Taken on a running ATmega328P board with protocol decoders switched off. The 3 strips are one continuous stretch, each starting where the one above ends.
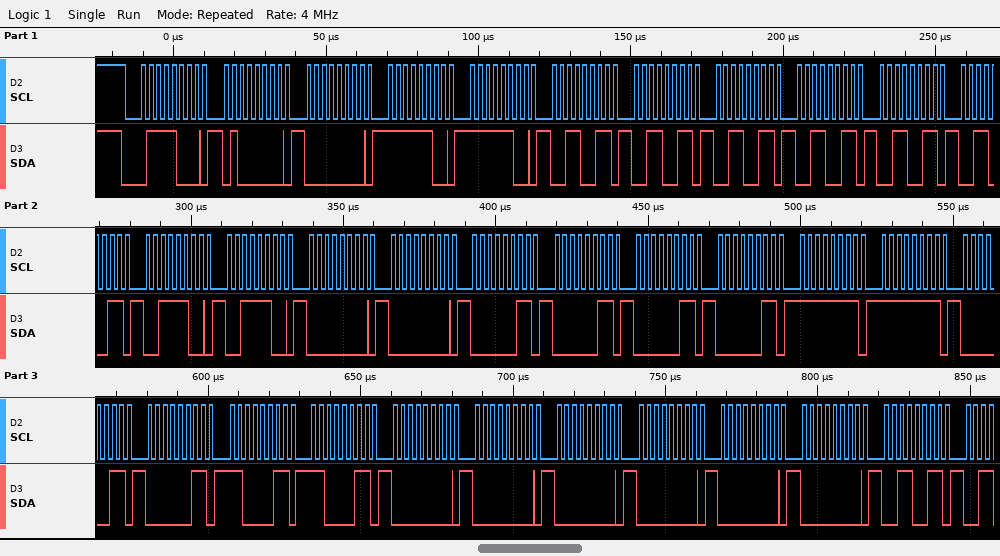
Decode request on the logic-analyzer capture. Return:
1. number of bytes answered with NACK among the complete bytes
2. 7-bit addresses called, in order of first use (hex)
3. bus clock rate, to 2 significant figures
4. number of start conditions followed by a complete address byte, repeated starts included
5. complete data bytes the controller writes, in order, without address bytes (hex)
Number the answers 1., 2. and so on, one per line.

1. 0
2. 0x3C
3. 400 kHz
4. 1
5. 40 00 FC FC 33 33 33 33 33 33 3C 3C 00 00 03 03 03 03 FF FF 03 03 C3 C3 00 00 00 00 00 00 33
